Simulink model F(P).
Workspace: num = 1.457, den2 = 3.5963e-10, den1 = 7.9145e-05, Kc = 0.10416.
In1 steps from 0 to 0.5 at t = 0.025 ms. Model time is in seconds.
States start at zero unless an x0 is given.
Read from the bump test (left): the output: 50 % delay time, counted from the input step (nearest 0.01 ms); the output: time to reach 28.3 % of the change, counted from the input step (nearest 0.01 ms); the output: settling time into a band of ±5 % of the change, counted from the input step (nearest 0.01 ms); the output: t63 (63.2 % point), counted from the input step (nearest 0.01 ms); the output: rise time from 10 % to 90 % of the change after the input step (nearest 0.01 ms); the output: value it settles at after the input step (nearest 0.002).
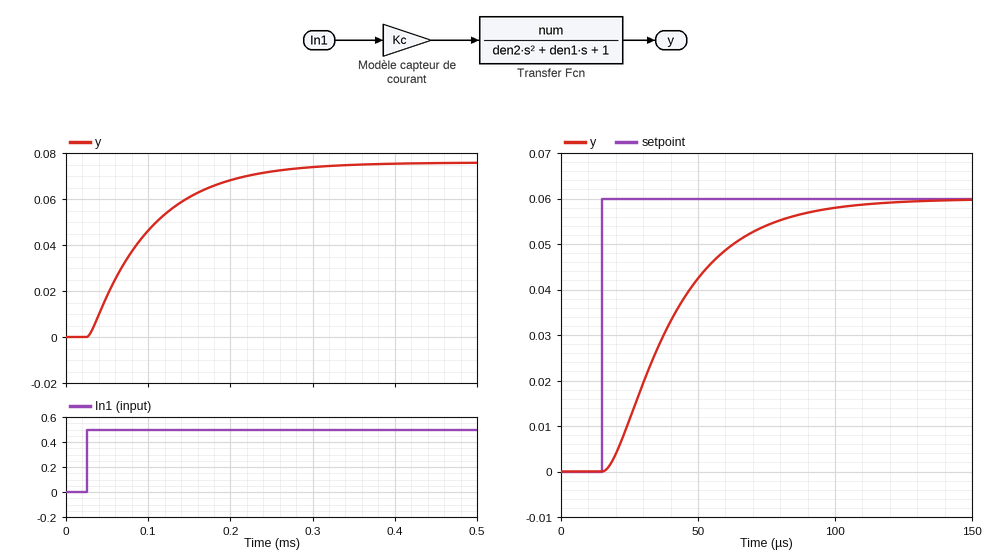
0.06 ms
0.03 ms
0.23 ms
0.08 ms
0.16 ms
0.076
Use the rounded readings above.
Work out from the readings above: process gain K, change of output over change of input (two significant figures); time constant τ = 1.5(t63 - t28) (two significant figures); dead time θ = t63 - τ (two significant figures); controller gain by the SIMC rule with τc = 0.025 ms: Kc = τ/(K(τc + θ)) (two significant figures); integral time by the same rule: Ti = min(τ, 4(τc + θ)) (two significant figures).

0.15
0.075 ms
0.0050 ms
17
0.075 ms
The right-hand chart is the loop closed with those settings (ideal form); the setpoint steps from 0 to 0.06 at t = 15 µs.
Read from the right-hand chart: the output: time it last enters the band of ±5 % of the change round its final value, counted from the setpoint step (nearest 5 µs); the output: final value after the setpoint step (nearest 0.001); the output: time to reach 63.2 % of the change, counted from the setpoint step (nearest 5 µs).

75 µs
0.060
30 µs
